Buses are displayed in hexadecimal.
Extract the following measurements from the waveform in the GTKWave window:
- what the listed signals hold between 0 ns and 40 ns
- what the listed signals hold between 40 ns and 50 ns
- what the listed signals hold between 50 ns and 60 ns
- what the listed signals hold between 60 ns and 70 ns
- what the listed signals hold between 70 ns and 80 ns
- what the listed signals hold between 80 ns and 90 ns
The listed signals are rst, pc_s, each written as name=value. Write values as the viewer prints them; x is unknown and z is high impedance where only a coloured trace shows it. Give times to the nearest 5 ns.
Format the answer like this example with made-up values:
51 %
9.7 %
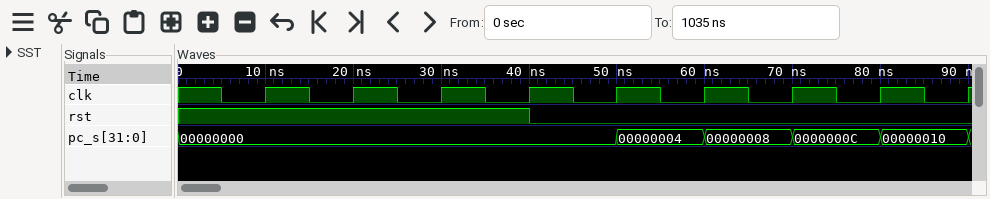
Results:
rst=1, pc_s=00000000
rst=0, pc_s=00000000
rst=0, pc_s=00000004
rst=0, pc_s=00000008
rst=0, pc_s=0000000C
rst=0, pc_s=00000010
